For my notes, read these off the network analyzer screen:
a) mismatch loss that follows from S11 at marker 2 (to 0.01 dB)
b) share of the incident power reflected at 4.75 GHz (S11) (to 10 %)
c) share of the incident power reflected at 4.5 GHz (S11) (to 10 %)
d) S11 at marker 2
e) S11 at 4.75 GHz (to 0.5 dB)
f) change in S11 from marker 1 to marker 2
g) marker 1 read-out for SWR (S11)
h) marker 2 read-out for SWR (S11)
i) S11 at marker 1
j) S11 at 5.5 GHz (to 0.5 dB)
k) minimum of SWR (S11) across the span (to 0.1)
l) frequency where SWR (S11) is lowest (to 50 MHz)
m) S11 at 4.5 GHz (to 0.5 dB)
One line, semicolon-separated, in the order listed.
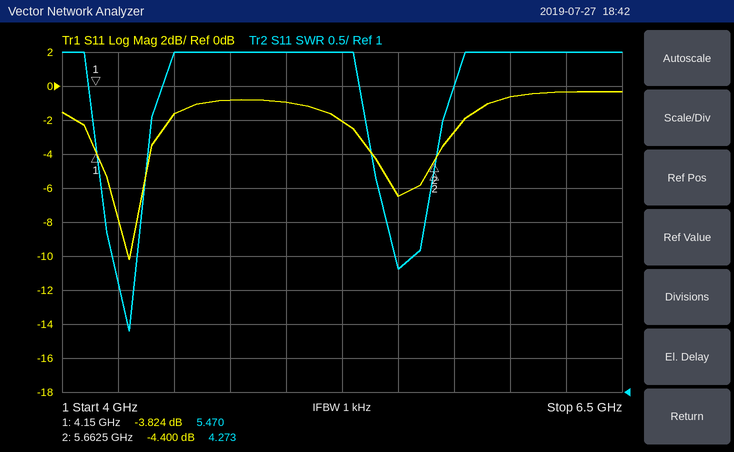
1.96 dB; 80 %; 70 %; -4.400 dB; -1.0 dB; -0.576 dB; 5.470; 4.273; -3.824 dB; -6.5 dB; 1.9; 4.30 GHz; -1.5 dB
